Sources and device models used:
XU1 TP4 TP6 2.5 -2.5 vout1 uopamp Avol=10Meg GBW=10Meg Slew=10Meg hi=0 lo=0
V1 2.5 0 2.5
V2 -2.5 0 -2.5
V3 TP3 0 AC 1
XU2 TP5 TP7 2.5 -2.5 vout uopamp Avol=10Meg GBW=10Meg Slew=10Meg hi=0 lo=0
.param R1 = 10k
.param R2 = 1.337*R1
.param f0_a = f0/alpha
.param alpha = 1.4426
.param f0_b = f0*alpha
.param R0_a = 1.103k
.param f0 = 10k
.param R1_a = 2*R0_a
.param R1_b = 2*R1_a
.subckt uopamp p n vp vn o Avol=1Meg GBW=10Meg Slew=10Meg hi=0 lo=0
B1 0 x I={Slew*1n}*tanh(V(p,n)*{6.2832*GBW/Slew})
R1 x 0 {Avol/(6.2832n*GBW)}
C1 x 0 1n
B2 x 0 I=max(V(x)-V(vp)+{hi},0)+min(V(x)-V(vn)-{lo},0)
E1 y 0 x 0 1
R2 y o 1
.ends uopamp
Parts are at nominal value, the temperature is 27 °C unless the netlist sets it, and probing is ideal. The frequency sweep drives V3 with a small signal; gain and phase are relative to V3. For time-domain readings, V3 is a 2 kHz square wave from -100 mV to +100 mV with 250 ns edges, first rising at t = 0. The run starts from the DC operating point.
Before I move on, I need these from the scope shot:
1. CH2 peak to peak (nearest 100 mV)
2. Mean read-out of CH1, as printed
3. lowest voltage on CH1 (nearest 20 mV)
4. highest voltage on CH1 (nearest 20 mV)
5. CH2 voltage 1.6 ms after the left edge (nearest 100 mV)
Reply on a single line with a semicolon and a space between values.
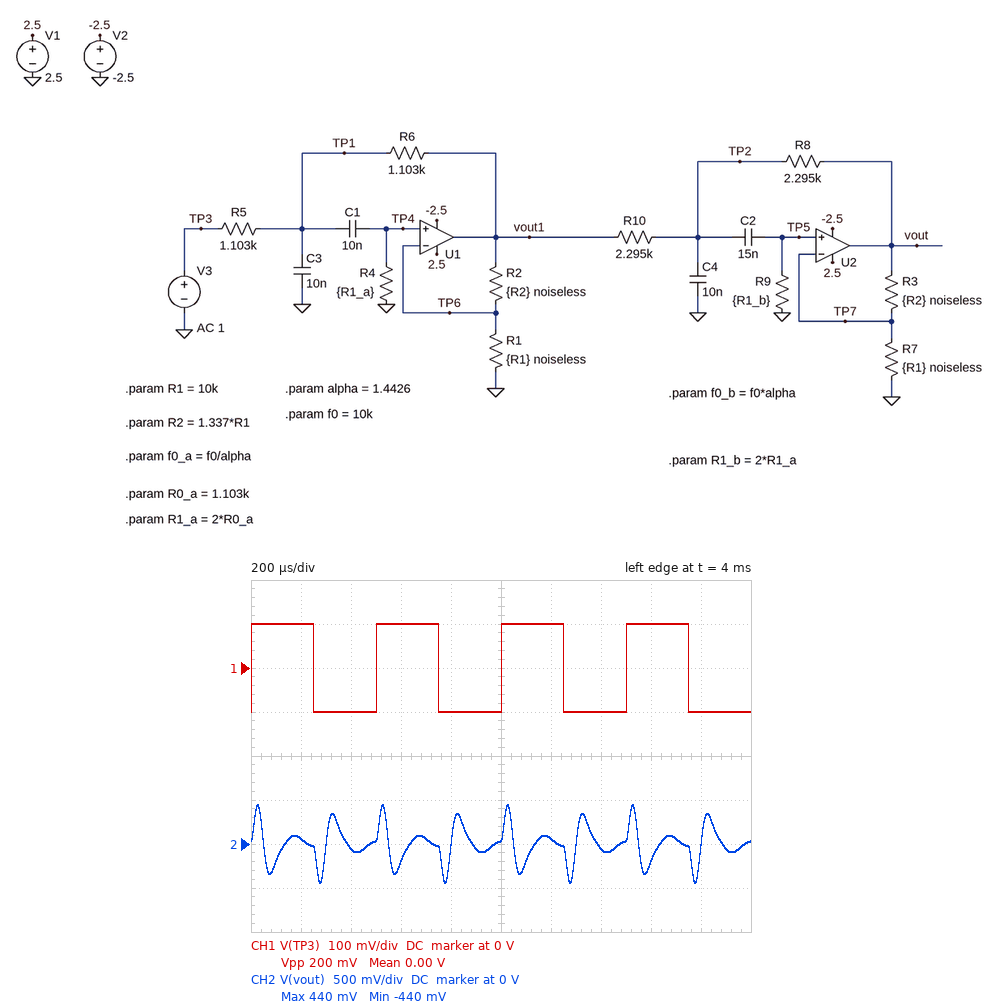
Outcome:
900 mV; 0.00 V; -100 mV; 100 mV; -200 mV
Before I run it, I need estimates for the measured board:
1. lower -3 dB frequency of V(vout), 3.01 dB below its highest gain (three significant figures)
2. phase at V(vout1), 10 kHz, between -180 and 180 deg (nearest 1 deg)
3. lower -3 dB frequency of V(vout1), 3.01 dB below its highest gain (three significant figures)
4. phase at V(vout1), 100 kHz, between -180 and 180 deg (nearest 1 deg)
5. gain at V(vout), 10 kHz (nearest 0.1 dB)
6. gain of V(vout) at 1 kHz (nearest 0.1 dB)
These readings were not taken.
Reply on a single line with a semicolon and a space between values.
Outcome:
5.03 kHz; 48 deg; 10.4 kHz; -86 deg; 13.9 dB; -21.8 dB
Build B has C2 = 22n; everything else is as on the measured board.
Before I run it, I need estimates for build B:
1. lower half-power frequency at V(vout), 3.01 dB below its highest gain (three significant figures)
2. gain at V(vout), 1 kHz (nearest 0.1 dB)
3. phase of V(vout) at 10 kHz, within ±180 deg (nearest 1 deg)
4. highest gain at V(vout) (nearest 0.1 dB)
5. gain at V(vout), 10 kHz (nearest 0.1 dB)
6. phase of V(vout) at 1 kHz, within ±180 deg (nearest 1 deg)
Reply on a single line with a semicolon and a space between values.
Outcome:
4.11 kHz; -18.4 dB; -21 deg; 14.0 dB; 13.2 dB; 170 deg
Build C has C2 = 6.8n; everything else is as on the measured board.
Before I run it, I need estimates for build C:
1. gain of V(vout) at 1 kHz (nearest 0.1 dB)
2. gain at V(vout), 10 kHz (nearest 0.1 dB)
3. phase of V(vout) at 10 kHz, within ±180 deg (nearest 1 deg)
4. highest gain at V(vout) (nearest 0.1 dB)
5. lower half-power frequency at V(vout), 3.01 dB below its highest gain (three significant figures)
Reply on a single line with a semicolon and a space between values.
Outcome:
-28.8 dB; 14.6 dB; 26 deg; 15.1 dB; 7.98 kHz
